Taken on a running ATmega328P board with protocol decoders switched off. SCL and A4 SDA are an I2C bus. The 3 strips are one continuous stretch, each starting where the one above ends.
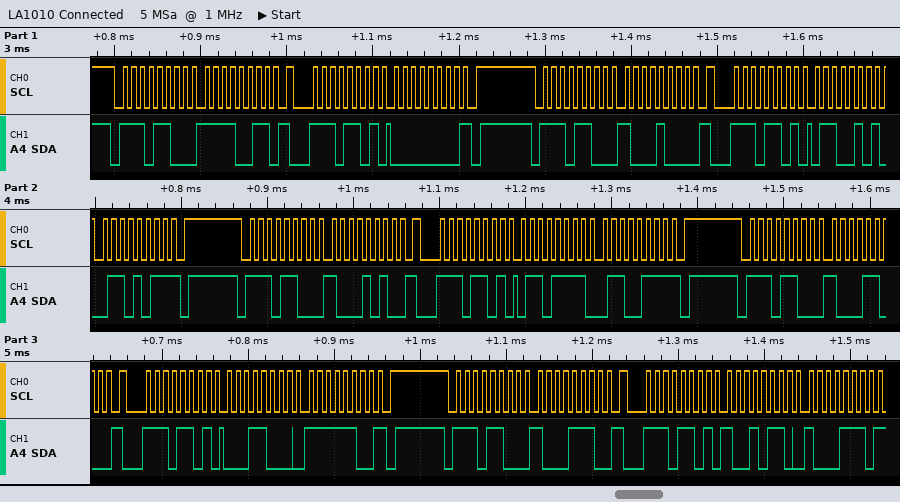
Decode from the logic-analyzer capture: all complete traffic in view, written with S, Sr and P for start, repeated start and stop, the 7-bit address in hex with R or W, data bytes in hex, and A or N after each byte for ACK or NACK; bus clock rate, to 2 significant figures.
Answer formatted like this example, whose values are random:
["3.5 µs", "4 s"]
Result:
["S 76W A F3 A Sr 76R A 00 N P S 76W A 88 A Sr 76R A 65 A 6B N P S 76W A 8A A Sr 76R A 6F A 67 N P S 76W A 8C A Sr 76R A 18 A FC N P S 76W A 8E A Sr 76R A 96 A 8E N", "100 kHz"]
